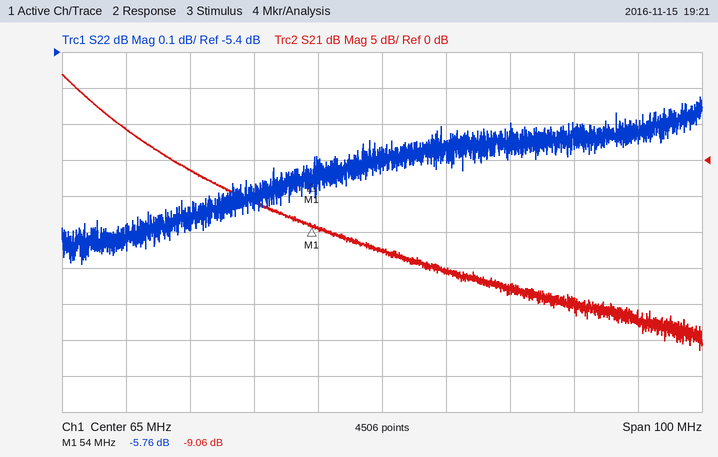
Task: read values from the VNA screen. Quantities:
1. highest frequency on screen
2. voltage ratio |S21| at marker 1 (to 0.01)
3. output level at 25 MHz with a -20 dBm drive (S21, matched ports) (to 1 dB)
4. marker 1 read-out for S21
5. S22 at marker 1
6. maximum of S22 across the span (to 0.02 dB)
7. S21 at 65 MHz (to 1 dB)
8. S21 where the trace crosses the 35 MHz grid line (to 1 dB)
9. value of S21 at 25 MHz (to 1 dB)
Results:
115 MHz
0.35
-16 dBm
-9.06 dB
-5.76 dB
-5.52 dB
-13 dB
-1 dB
4 dB
